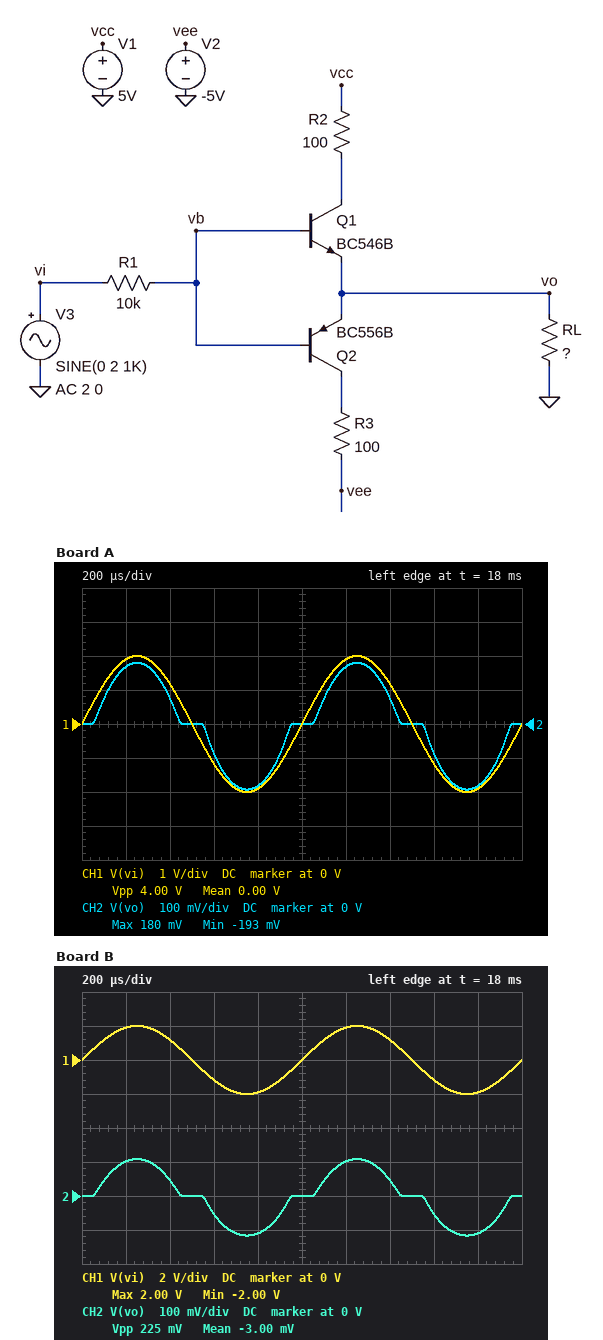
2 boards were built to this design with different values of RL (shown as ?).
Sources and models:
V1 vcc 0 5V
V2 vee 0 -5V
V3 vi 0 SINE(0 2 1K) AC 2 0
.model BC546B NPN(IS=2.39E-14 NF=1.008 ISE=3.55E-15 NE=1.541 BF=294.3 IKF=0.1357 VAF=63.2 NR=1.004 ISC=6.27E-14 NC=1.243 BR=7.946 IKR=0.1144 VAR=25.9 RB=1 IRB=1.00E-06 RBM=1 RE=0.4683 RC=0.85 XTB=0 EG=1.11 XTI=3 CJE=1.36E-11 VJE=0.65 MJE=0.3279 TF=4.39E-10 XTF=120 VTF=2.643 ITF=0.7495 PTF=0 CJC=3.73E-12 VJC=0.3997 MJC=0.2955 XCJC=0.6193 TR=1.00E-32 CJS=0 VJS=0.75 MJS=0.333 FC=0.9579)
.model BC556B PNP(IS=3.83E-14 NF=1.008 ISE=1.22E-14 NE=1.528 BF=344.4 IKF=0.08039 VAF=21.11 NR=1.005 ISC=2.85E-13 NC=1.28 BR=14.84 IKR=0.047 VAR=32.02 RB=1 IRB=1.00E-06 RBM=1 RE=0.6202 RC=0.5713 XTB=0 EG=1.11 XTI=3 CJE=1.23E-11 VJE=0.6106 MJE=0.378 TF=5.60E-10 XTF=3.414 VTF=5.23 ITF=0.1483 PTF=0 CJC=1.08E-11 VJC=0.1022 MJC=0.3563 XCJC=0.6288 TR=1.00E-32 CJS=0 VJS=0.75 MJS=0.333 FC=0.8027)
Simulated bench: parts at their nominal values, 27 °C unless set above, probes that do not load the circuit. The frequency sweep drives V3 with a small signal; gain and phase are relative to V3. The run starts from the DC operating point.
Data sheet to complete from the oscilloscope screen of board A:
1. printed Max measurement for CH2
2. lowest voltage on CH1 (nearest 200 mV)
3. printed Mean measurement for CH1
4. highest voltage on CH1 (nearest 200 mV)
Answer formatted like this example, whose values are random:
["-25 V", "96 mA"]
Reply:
["180 mV", "-2.0 V", "0.00 V", "2.0 V"]
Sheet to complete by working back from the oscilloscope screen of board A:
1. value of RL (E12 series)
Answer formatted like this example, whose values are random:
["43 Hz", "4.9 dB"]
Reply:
["6.8 Ω"]
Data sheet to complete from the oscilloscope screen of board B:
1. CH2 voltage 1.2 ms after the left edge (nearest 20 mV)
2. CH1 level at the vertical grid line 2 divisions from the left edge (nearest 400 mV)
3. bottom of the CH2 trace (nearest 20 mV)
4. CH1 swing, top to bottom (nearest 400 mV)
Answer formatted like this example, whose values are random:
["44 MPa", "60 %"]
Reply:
["100 mV", "1.2 V", "-120 mV", "4.0 V"]
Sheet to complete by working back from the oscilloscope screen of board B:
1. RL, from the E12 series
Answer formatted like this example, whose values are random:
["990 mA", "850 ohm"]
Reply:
["3.9 Ω"]
